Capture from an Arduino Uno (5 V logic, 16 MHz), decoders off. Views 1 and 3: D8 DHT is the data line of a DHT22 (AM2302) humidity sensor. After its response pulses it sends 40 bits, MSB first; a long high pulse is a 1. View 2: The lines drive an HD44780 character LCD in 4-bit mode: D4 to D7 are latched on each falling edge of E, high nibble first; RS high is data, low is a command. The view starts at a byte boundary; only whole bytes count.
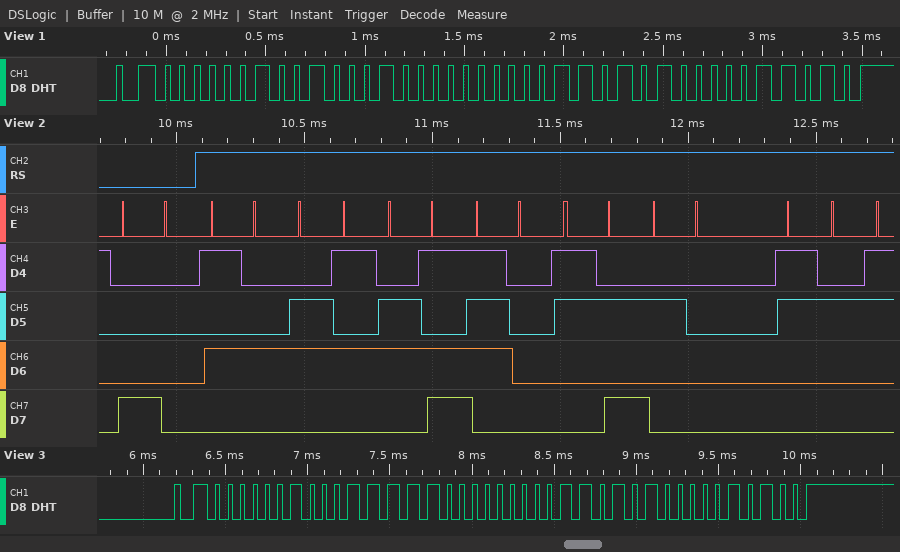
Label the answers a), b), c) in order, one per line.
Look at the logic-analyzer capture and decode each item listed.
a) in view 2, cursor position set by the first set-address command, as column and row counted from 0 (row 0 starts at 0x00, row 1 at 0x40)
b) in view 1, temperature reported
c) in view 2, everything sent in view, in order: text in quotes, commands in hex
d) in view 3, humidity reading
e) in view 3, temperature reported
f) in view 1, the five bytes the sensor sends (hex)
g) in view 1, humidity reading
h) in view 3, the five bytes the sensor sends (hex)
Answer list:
a) column 0, row 0
b) 21.2 °C
c) 0x80 "Temp: 2"
d) 57.4 %
e) 21.2 °C
f) 02 44 00 D4 1A
g) 58.0 %
h) 02 3E 00 D4 14
